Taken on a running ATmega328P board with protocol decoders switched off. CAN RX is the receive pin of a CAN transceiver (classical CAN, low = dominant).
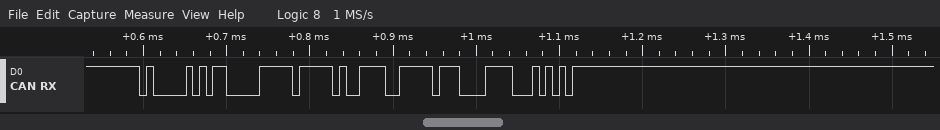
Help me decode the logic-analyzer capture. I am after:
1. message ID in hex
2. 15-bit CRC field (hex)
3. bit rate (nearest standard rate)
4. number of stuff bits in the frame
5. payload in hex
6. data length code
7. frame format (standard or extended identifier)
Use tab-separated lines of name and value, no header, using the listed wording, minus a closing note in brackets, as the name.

message ID in hex	0x40B
15-bit CRC field	0x078A
bit rate	125 kbit/s
number of stuff bits in the frame	5
payload in hex	FF 3C FF
data length code	3
frame format	standard
